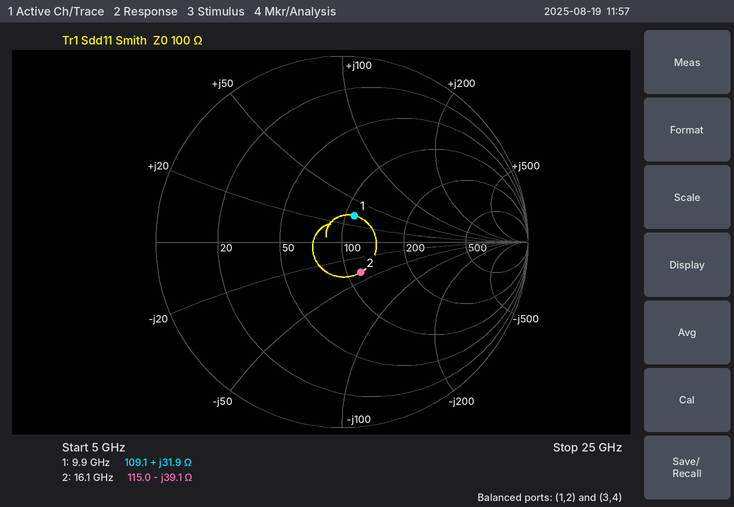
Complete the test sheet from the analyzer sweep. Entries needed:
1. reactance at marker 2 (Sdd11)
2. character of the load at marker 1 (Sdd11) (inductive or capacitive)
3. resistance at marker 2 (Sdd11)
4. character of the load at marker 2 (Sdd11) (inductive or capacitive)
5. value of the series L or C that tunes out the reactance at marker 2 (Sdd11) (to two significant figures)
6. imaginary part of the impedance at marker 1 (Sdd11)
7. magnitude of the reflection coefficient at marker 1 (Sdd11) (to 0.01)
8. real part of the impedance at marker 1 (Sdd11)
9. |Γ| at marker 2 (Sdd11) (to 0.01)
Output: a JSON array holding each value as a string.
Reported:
["-39.1 Ω", "inductive", "115.0 Ω", "capacitive", "390 pH", "+31.9 Ω", "0.16", "109.1 Ω", "0.19"]
